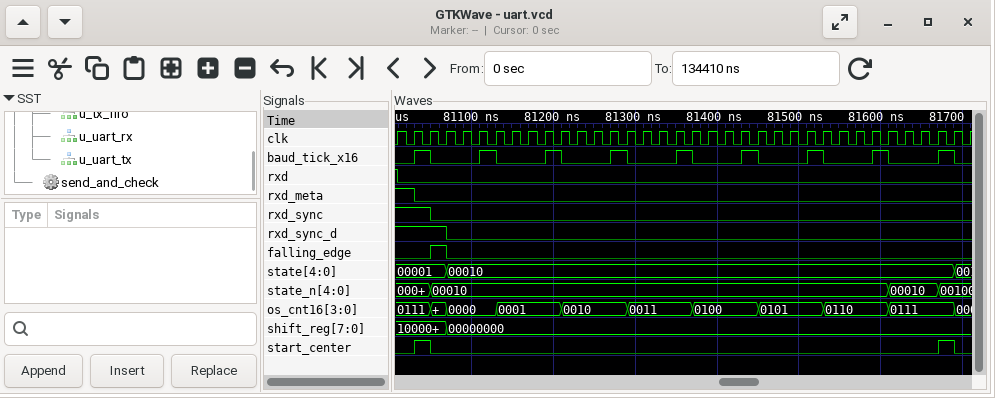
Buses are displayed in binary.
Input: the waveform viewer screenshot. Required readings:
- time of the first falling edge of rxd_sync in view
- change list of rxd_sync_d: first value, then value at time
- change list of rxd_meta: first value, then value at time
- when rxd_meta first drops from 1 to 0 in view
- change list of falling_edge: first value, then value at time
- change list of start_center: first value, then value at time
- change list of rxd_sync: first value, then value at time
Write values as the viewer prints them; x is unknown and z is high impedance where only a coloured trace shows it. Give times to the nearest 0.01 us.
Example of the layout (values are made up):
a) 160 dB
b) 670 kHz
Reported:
a) 81.05 us
b) 1, 0 at 81.07 us
c) 1, 0 at 81.03 us
d) 81.03 us
e) 0, 1 at 81.05 us, 0 at 81.07 us
f) 0, 1 at 81.03 us, 0 at 81.05 us, 1 at 81.67 us, 0 at 81.69 us
g) 1, 0 at 81.05 us
